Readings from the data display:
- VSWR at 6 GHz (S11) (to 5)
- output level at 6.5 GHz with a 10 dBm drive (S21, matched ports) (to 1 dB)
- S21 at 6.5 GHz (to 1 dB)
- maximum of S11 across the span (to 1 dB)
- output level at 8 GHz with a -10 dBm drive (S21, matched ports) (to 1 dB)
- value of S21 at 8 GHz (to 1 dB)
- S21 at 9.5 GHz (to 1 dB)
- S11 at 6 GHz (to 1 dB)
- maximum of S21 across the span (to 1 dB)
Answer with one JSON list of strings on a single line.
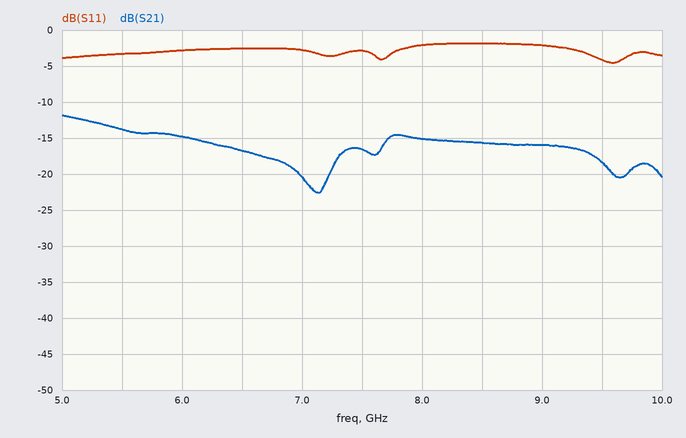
["5", "-7 dBm", "-17 dB", "-2 dB", "-25 dBm", "-15 dB", "-18 dB", "-3 dB", "-12 dB"]
